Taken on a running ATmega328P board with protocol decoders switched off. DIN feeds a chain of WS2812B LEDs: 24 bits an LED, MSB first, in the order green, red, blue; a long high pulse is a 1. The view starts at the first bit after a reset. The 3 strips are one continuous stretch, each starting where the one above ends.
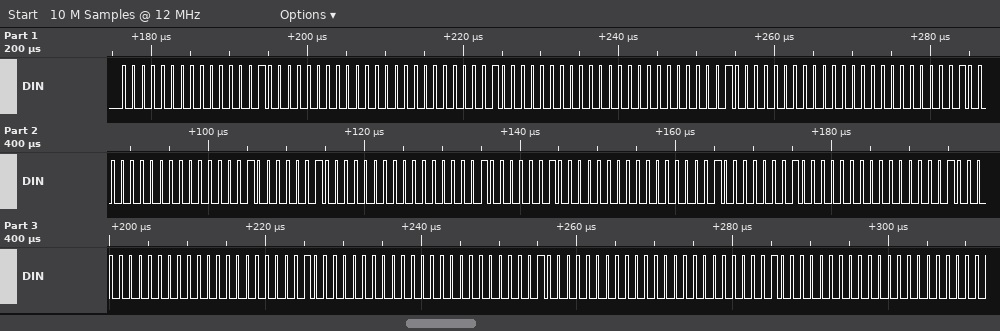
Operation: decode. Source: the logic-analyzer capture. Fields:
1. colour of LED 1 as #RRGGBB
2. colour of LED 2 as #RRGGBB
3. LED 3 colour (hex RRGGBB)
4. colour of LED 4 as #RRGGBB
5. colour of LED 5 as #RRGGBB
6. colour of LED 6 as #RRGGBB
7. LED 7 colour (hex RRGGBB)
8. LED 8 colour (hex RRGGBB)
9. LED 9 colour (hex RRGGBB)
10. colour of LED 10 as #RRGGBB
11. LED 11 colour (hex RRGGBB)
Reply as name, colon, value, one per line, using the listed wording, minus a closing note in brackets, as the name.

colour of LED 1 as #RRGGBB: #020000
colour of LED 2 as #RRGGBB: #020000
LED 3 colour: #020000
colour of LED 4 as #RRGGBB: #020000
colour of LED 5 as #RRGGBB: #020100
colour of LED 6 as #RRGGBB: #020100
LED 7 colour: #010100
LED 8 colour: #000100
LED 9 colour: #000100
colour of LED 10 as #RRGGBB: #000100
LED 11 colour: #000100
